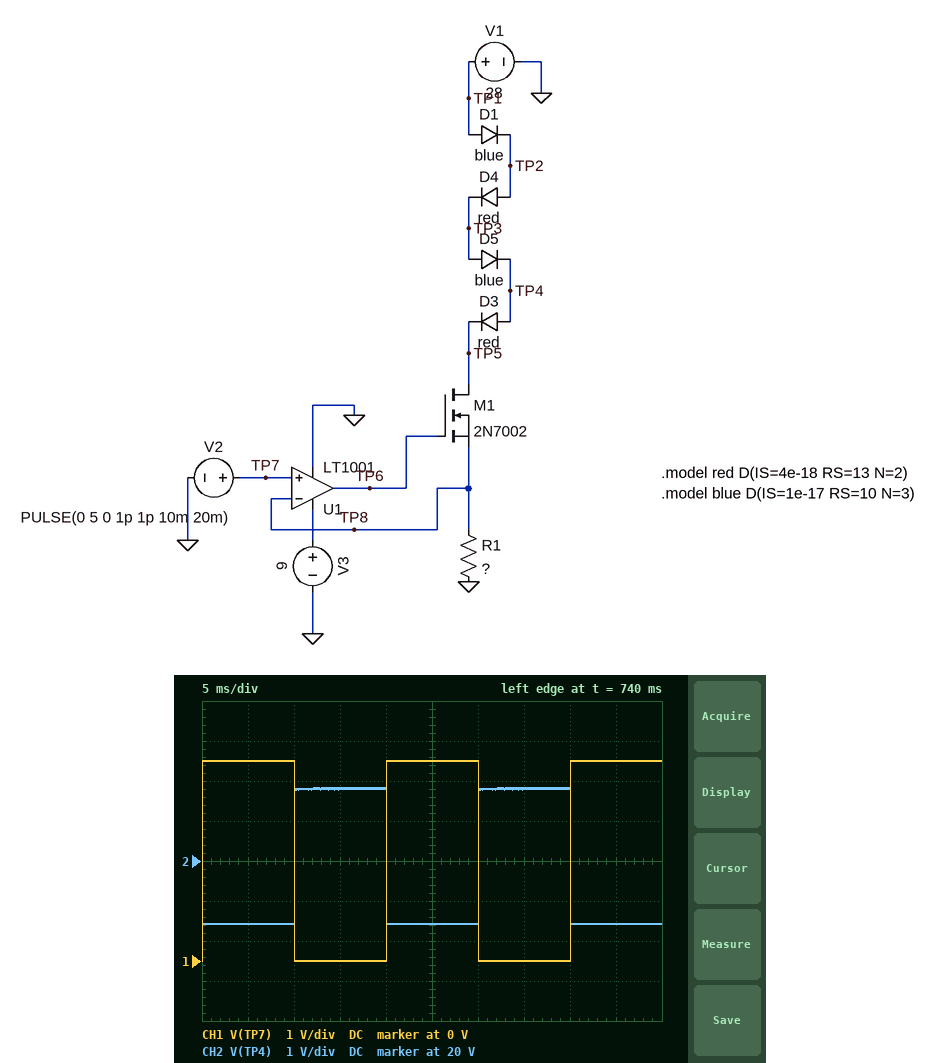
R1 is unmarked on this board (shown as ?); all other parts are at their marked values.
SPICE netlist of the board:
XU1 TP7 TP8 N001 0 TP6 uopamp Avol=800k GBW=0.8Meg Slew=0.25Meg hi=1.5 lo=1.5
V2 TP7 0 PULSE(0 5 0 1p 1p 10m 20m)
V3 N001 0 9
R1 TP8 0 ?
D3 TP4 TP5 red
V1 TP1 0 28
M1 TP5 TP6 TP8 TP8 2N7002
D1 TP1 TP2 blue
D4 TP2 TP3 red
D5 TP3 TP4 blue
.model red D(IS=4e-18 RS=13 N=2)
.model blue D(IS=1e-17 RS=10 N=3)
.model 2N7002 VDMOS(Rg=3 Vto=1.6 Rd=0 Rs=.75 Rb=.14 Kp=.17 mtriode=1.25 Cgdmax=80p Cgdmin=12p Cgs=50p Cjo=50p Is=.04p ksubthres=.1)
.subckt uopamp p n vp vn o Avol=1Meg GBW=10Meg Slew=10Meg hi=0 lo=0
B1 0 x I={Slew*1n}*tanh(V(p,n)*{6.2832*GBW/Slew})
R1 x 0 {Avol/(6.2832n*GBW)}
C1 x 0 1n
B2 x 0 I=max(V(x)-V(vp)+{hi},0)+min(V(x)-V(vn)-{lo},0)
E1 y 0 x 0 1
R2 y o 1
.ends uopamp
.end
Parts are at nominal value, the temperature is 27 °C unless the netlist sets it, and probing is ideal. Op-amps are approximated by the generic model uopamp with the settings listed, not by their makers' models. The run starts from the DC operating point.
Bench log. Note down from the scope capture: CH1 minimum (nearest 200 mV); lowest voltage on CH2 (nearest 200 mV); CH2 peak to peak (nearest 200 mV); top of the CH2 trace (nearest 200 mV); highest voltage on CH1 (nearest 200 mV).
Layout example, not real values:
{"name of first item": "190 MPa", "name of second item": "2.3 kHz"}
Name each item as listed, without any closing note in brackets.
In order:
{"CH1 minimum": "0 V", "lowest voltage on CH2": "18.4 V", "CH2 peak to peak": "3.4 V", "top of the CH2 trace": "21.8 V", "highest voltage on CH1": "5.0 V"}
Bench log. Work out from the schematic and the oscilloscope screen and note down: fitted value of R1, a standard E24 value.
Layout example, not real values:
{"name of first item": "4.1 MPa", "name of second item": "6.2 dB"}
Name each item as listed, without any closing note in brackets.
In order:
{"fitted value of R1, a standard E24 value": "82 Ω"}
